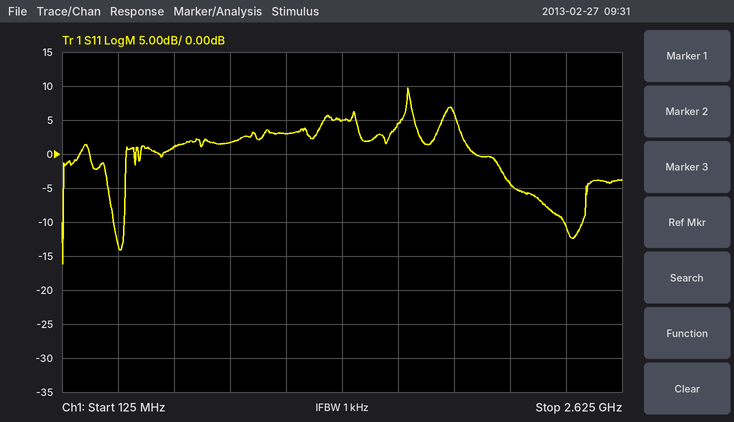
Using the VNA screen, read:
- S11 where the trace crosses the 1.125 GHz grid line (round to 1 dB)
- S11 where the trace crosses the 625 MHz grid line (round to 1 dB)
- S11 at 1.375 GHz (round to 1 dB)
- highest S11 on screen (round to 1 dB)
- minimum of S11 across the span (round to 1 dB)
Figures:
3 dB
1 dB
5 dB
10 dB
-16 dB
